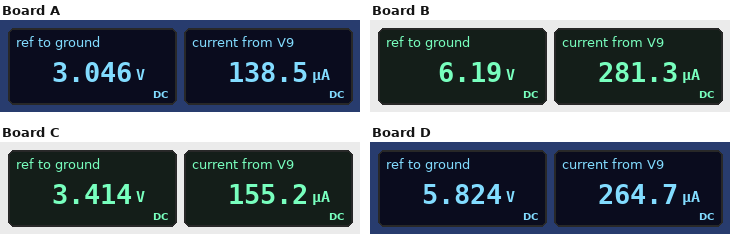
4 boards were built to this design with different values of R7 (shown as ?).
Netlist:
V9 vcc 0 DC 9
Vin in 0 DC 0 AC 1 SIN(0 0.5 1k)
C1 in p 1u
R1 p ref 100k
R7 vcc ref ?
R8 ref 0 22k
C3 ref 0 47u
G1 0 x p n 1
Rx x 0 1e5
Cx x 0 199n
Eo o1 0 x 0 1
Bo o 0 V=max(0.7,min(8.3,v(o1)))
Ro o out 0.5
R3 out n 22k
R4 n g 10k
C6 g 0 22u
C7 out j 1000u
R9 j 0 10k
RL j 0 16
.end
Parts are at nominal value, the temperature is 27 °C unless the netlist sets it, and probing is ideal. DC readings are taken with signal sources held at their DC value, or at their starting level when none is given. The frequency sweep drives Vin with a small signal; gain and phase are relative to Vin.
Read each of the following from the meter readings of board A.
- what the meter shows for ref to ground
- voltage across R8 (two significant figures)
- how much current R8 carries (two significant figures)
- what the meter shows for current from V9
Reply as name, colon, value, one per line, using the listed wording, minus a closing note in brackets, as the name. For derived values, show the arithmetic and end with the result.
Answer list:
what the meter shows for ref to ground: 3.046 V
voltage across R8: 3.046 V = 3.0 V
how much current R8 carries: (3.046 V) / 22 kΩ = 140 µA
what the meter shows for current from V9: 138.5 µA
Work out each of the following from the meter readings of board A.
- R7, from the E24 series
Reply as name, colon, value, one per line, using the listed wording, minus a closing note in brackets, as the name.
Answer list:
R7, from the E24 series: 43 kΩ
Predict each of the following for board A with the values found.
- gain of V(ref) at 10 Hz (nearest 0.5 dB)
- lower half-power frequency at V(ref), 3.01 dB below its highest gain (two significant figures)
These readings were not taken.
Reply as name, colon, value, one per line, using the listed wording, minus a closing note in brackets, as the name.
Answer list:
gain of V(ref) at 10 Hz: -49.5 dB
lower half-power frequency at V(ref), 3.01 dB below its highest gain: 180 mHz
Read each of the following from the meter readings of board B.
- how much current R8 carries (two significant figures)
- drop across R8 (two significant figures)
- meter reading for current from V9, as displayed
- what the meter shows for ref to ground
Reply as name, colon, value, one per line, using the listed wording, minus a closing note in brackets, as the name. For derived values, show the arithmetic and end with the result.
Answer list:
how much current R8 carries: (6.19 V) / 22 kΩ = 280 µA
drop across R8: 6.19 V = 6.2 V
meter reading for current from V9, as displayed: 281.3 µA
what the meter shows for ref to ground: 6.19 V
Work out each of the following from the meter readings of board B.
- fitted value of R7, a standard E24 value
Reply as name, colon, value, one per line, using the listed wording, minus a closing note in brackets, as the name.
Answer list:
fitted value of R7, a standard E24 value: 10 kΩ
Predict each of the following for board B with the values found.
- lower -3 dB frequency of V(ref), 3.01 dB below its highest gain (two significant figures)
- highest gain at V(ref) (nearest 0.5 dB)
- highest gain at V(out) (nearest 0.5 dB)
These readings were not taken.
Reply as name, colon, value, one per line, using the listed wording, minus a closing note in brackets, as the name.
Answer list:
lower -3 dB frequency of V(ref), 3.01 dB below its highest gain: 320 mHz
highest gain at V(ref): -36.0 dB
highest gain at V(out): 10.0 dB
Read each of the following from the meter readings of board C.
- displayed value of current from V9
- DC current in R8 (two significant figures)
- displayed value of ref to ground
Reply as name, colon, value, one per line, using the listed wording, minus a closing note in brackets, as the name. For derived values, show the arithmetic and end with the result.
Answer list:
displayed value of current from V9: 155.2 µA
DC current in R8: (3.414 V) / 22 kΩ = 160 µA
displayed value of ref to ground: 3.414 V
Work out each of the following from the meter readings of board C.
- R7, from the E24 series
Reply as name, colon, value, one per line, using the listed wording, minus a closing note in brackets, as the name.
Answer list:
R7, from the E24 series: 36 kΩ
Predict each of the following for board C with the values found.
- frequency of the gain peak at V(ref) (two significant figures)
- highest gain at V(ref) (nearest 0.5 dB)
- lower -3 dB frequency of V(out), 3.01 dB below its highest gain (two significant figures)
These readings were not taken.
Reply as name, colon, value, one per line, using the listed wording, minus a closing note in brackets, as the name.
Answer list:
frequency of the gain peak at V(ref): 630 mHz
highest gain at V(ref): -35.0 dB
lower -3 dB frequency of V(out), 3.01 dB below its highest gain: 1.9 Hz
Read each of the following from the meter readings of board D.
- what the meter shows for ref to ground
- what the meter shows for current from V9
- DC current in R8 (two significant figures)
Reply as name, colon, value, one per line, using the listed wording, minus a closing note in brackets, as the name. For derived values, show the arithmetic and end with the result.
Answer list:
what the meter shows for ref to ground: 5.824 V
what the meter shows for current from V9: 264.7 µA
DC current in R8: (5.824 V) / 22 kΩ = 260 µA
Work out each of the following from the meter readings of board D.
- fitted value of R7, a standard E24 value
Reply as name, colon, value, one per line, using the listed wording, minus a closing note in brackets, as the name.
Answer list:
fitted value of R7, a standard E24 value: 12 kΩ
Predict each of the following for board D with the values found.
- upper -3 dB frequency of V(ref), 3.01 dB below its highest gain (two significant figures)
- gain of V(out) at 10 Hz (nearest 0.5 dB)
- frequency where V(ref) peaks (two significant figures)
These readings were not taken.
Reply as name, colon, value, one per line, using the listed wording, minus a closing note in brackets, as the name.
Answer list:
upper -3 dB frequency of V(ref), 3.01 dB below its highest gain: 2.4 Hz
gain of V(out) at 10 Hz: 10.0 dB
frequency where V(ref) peaks: 830 mHz
